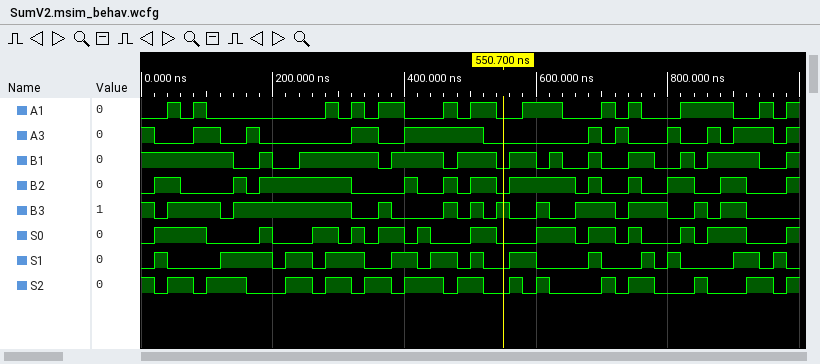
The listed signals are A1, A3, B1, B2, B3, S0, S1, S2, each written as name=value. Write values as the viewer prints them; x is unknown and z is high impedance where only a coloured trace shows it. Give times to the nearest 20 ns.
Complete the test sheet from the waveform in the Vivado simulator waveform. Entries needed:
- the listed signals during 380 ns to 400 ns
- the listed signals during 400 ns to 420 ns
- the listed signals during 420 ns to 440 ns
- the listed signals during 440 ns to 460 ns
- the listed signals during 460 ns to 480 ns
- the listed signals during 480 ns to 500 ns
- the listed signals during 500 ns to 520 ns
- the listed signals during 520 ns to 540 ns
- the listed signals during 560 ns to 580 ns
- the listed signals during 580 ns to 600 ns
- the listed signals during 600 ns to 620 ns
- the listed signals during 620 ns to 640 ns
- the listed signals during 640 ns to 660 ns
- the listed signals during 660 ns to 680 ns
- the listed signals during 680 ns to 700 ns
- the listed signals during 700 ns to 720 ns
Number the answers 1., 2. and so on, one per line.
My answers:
1. A1=1, A3=0, B1=1, B2=0, B3=0, S0=1, S1=1, S2=0
2. A1=0, A3=1, B1=1, B2=1, B3=0, S0=0, S1=1, S2=1
3. A1=0, A3=1, B1=1, B2=0, B3=0, S0=1, S1=0, S2=1
4. A1=0, A3=1, B1=1, B2=0, B3=0, S0=0, S1=1, S2=1
5. A1=1, A3=1, B1=0, B2=1, B3=1, S0=0, S1=1, S2=0
6. A1=0, A3=1, B1=1, B2=0, B3=0, S0=0, S1=0, S2=1
7. A1=1, A3=1, B1=1, B2=1, B3=1, S0=1, S1=1, S2=1
8. A1=1, A3=0, B1=1, B2=1, B3=0, S0=1, S1=0, S2=0
9. A1=0, A3=0, B1=1, B2=1, B3=0, S0=0, S1=1, S2=1
10. A1=1, A3=0, B1=1, B2=1, B3=0, S0=0, S1=1, S2=0
11. A1=1, A3=0, B1=0, B2=1, B3=1, S0=1, S1=0, S2=1
12. A1=1, A3=0, B1=1, B2=1, B3=0, S0=1, S1=0, S2=0
13. A1=0, A3=0, B1=0, B2=1, B3=0, S0=1, S1=0, S2=0
14. A1=0, A3=0, B1=0, B2=0, B3=1, S0=0, S1=0, S2=0
15. A1=0, A3=1, B1=1, B2=1, B3=1, S0=1, S1=1, S2=0
16. A1=1, A3=0, B1=0, B2=0, B3=1, S0=1, S1=0, S2=1
